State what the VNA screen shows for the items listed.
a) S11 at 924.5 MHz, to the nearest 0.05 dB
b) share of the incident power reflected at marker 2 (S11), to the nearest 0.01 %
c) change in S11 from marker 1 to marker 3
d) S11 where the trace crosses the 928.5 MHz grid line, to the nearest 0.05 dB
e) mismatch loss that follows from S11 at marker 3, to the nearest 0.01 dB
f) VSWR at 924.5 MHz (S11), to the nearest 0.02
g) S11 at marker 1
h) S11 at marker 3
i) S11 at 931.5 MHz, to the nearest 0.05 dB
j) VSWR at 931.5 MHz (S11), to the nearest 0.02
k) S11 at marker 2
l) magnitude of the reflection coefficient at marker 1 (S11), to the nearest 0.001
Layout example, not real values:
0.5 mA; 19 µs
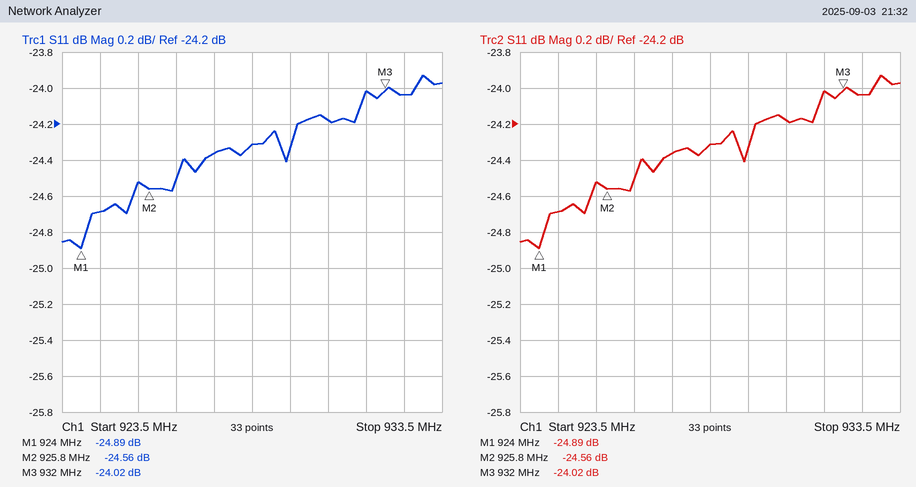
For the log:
-24.70 dB; 0.35 %; 0.87 dB; -24.30 dB; 0.02 dB; 1.12; -24.89 dB; -24.02 dB; -24.00 dB; 1.14; -24.56 dB; 0.057
